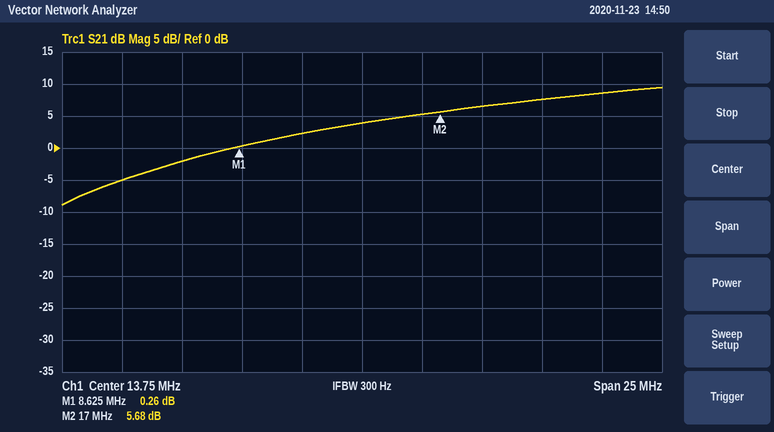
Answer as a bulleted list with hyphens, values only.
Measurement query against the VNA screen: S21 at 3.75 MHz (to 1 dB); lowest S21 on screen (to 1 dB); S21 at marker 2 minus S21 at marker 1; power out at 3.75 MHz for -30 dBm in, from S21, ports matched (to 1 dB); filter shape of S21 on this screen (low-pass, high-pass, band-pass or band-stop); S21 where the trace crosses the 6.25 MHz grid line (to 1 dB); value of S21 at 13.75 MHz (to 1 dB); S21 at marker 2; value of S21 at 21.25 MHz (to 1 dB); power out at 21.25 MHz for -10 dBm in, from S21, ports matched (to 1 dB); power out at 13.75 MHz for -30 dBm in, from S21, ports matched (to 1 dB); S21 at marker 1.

- -5 dB
- -9 dB
- 5.42 dB
- -35 dBm
- high-pass
- -2 dB
- 4 dB
- 5.68 dB
- 8 dB
- -2 dBm
- -26 dBm
- 0.26 dB
